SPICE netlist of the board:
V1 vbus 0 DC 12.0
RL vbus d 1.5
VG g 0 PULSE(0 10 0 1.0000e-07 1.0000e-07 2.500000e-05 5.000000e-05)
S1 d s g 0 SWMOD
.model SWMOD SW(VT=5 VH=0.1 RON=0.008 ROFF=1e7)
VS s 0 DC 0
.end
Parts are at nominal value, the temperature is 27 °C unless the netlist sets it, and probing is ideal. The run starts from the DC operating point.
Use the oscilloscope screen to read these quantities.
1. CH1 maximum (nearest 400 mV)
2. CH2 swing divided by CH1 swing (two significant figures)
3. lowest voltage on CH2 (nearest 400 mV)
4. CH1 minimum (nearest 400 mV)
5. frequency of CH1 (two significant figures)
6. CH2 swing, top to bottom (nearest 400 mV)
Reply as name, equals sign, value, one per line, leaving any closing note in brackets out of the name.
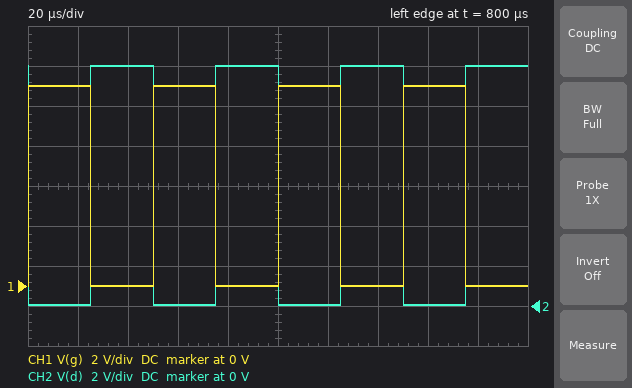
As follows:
CH1 maximum = 10.0 V
CH2 swing divided by CH1 swing = 1.2
lowest voltage on CH2 = 0 V
CH1 minimum = 0 V
frequency of CH1 = 20 kHz
CH2 swing, top to bottom = 12.0 V
